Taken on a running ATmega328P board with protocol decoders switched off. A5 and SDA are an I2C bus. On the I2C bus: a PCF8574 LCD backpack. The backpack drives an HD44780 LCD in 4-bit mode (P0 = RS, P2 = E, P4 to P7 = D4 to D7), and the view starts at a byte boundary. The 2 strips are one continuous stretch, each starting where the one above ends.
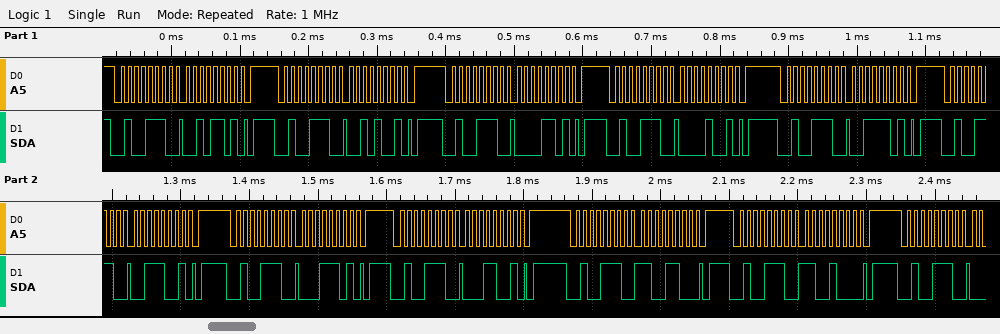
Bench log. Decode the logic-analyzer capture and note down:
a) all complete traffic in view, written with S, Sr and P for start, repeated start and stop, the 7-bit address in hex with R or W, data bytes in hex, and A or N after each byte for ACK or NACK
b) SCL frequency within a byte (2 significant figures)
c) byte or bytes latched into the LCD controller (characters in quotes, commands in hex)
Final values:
S 27W A 2D A P S 27W A 29 A P S 27W A 0D A P S 27W A 09 A P S 27W A 3D A P S 27W A 39 A P S 27W A 1D A P S 27W A 19 A P S 27W A CC A P S 27W A C8 A P S 27W A
100 kHz
' ' '1'
